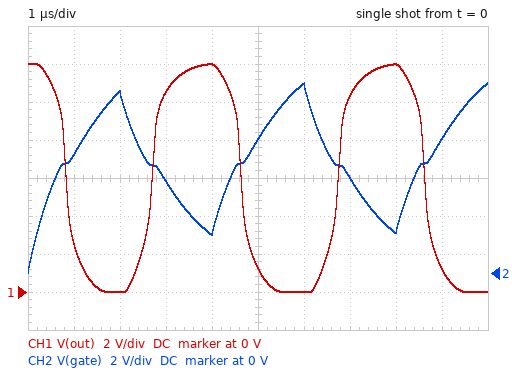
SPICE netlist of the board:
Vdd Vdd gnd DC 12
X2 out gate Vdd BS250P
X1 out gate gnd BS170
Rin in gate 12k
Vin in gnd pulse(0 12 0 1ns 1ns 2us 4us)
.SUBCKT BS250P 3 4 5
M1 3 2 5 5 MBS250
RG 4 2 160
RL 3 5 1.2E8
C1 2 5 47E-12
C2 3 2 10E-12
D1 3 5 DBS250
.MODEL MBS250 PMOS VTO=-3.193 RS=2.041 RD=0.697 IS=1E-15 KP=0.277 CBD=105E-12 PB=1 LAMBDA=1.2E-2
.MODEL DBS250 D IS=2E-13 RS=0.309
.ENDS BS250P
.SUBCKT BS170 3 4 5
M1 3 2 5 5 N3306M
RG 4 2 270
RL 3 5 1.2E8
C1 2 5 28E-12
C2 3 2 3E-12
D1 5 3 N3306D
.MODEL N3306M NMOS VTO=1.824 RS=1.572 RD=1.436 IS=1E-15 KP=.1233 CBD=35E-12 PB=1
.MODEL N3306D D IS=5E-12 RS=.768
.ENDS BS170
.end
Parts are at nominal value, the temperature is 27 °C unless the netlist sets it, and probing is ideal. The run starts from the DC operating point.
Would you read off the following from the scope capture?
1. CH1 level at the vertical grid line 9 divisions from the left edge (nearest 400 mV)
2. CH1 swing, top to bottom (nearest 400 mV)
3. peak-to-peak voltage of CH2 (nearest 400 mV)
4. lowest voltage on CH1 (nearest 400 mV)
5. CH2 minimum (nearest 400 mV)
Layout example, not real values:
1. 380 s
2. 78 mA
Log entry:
1. 1.2 V
2. 12.0 V
3. 10.0 V
4. 0 V
5. 0 V
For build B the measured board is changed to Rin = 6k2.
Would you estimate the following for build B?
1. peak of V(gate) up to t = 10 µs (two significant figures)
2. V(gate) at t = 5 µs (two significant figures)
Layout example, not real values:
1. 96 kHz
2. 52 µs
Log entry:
1. 12 V
2. 9.5 V
